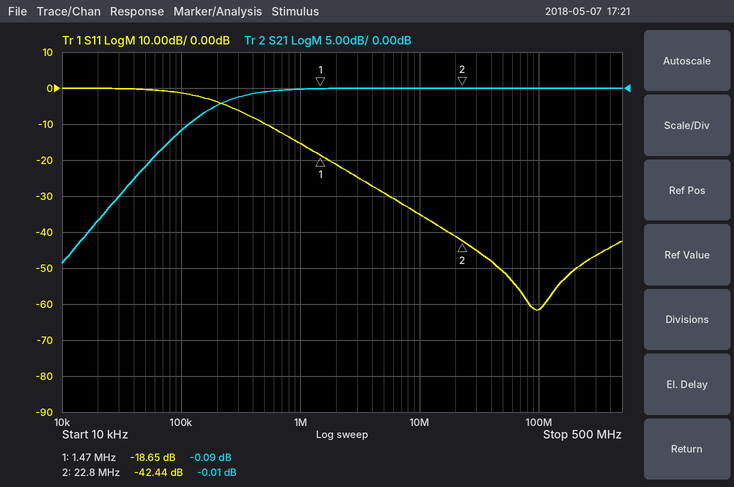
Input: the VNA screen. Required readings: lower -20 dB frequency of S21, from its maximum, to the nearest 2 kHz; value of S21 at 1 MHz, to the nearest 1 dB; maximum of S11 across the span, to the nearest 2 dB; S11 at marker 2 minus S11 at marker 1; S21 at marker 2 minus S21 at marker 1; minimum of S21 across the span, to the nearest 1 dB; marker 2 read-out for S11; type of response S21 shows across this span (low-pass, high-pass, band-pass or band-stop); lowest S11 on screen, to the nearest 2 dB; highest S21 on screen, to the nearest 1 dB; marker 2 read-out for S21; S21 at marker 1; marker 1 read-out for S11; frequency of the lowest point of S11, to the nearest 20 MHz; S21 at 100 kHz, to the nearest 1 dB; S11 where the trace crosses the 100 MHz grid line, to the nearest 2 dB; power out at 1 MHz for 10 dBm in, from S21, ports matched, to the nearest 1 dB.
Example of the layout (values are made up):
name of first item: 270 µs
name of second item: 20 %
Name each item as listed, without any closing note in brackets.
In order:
lower -20 dB frequency of S21, from its maximum, to the nearest 2 kHz: 16 kHz
value of S21 at 1 MHz, to the nearest 1 dB: 0 dB
maximum of S11 across the span, to the nearest 2 dB: 0 dB
S11 at marker 2 minus S11 at marker 1: -23.79 dB
S21 at marker 2 minus S21 at marker 1: 0.08 dB
minimum of S21 across the span, to the nearest 1 dB: -24 dB
marker 2 read-out for S11: -42.44 dB
type of response S21 shows across this span: high-pass
lowest S11 on screen, to the nearest 2 dB: -62 dB
highest S21 on screen, to the nearest 1 dB: 0 dB
marker 2 read-out for S21: -0.01 dB
S21 at marker 1: -0.09 dB
marker 1 read-out for S11: -18.65 dB
frequency of the lowest point of S11, to the nearest 20 MHz: 100 MHz
S21 at 100 kHz, to the nearest 1 dB: -6 dB
S11 where the trace crosses the 100 MHz grid line, to the nearest 2 dB: -62 dB
power out at 1 MHz for 10 dBm in, from S21, ports matched, to the nearest 1 dB: 10 dBm
